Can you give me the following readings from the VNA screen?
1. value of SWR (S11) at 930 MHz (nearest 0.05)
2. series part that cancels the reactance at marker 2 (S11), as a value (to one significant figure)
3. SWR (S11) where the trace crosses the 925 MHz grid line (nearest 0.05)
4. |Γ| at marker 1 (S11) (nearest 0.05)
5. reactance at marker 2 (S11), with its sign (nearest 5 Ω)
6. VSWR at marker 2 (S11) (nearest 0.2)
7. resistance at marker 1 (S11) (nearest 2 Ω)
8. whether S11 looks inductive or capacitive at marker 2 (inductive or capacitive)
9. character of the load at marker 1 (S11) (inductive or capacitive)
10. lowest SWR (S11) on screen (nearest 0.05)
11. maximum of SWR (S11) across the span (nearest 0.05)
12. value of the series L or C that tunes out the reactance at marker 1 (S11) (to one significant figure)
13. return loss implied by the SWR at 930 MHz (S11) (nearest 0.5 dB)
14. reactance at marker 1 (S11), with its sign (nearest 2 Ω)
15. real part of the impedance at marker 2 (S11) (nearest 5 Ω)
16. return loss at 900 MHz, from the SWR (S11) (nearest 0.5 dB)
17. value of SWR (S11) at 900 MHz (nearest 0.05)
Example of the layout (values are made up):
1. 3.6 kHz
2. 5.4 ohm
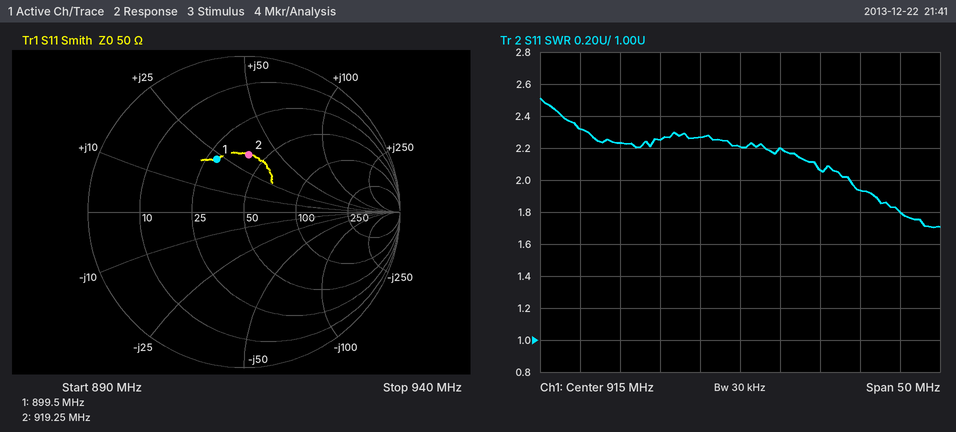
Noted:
1. 1.95
2. 5 pF
3. 2.05
4. 0.40
5. +35 Ω
6. 2.2
7. 28 Ω
8. inductive
9. inductive
10. 1.70
11. 2.50
12. 8 pF
13. 10.0 dB
14. +22 Ω
15. 40 Ω
16. 8.5 dB
17. 2.25
